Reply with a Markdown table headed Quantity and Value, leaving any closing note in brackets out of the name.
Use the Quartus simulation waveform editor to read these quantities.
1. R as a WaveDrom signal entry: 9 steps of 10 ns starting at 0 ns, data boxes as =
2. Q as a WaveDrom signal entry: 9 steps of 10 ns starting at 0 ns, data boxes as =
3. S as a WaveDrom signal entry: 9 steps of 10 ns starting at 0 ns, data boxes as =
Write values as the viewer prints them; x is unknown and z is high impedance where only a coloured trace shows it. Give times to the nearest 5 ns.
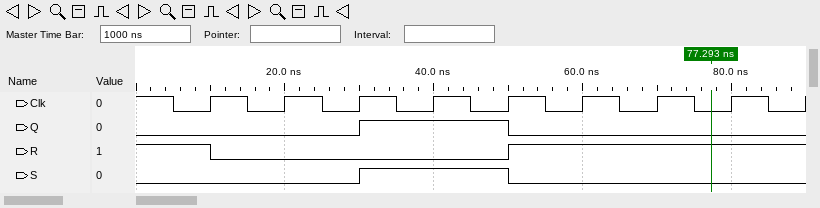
| Quantity | Value |
|---|---|
| R as a WaveDrom signal entry: 9 steps of 10 ns starting at 0 ns, data boxes as = | {name: 'R', wave: '10...1...'} |
| Q as a WaveDrom signal entry: 9 steps of 10 ns starting at 0 ns, data boxes as = | {name: 'Q', wave: '0..1.0...'} |
| S as a WaveDrom signal entry: 9 steps of 10 ns starting at 0 ns, data boxes as = | {name: 'S', wave: '0..1.0...'} |
